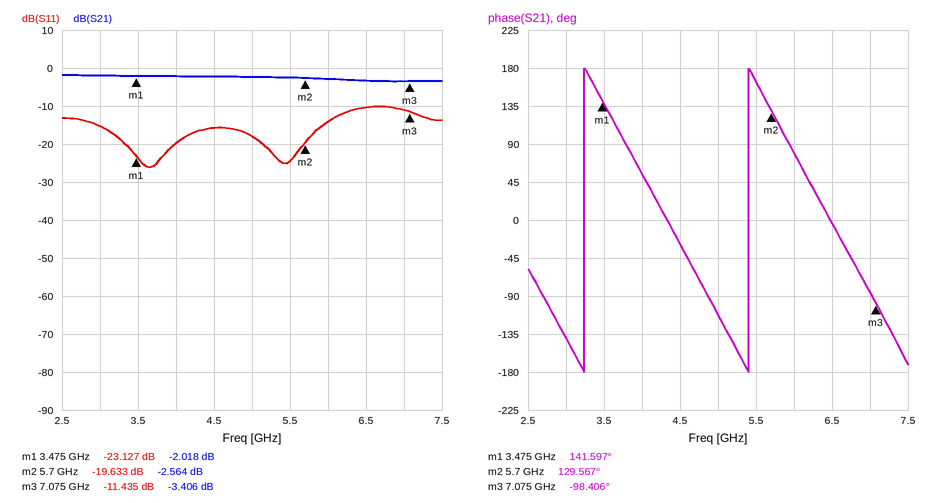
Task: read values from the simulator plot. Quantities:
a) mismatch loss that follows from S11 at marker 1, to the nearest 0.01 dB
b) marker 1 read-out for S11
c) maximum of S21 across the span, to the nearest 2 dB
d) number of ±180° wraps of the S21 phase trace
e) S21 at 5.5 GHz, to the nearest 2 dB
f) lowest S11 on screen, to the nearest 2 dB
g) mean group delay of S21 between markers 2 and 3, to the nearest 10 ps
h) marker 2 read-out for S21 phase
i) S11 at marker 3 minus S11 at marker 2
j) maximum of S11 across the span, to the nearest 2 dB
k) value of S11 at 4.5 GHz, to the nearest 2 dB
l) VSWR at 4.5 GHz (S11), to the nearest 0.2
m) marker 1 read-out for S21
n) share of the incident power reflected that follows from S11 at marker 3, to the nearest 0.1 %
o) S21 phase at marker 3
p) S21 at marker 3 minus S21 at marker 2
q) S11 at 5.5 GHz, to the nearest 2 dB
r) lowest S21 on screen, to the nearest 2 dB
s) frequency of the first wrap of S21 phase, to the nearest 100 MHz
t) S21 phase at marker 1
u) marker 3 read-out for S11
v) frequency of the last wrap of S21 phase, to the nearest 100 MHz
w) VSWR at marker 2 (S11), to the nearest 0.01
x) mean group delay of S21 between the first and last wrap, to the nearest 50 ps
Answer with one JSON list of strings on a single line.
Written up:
["0.02 dB", "-23.127 dB", "-2 dB", "2", "-2 dB", "-26 dB", "460 ps", "129.567°", "8.198 dB", "-10 dB", "-16 dB", "1.4", "-2.018 dB", "7.2 %", "-98.406°", "-0.842 dB", "-24 dB", "-4 dB", "3.2 GHz", "141.597°", "-11.435 dB", "5.4 GHz", "1.23", "450 ps"]
